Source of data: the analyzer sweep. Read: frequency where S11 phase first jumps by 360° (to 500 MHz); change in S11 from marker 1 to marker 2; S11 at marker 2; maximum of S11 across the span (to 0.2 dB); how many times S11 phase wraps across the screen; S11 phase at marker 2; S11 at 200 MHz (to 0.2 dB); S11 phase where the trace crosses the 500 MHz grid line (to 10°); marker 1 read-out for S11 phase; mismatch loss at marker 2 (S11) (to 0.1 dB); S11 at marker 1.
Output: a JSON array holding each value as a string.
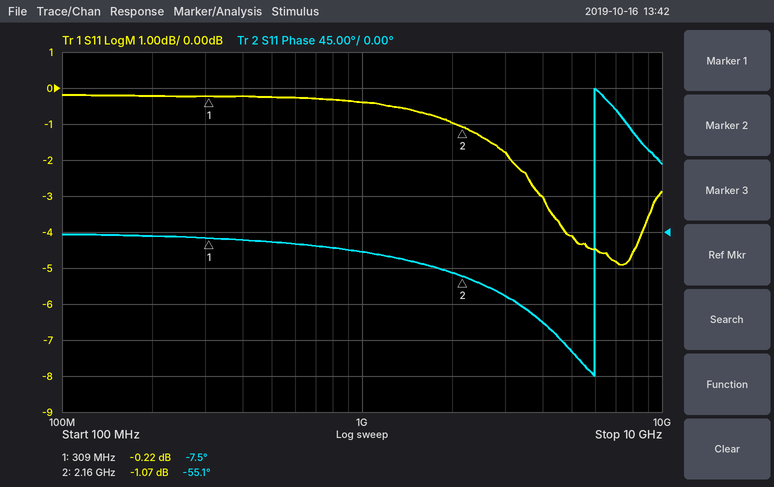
["6.0 GHz", "-0.85 dB", "-1.07 dB", "-0.2 dB", "1", "-55.1°", "-0.2 dB", "-10°", "-7.5°", "6.6 dB", "-0.22 dB"]
